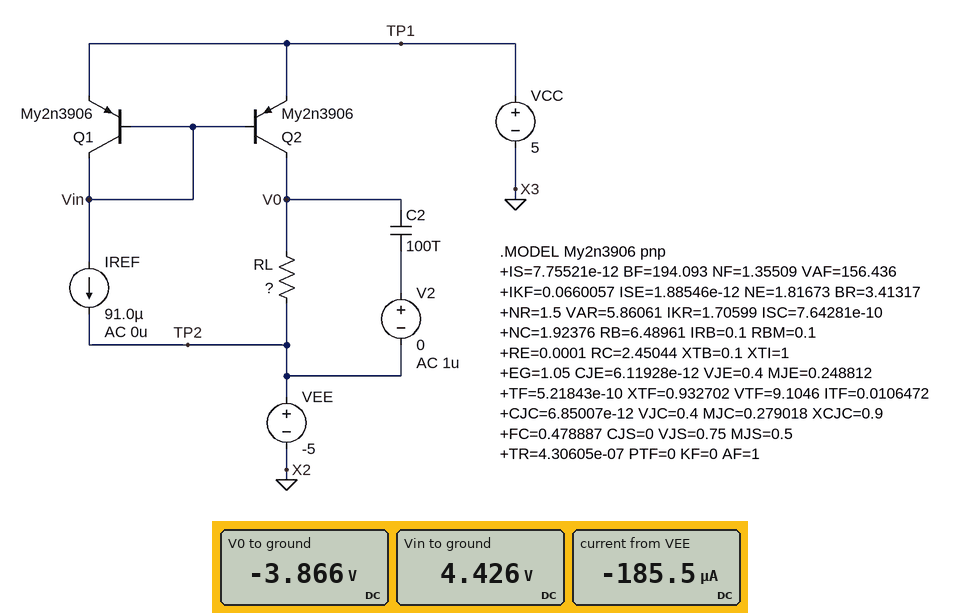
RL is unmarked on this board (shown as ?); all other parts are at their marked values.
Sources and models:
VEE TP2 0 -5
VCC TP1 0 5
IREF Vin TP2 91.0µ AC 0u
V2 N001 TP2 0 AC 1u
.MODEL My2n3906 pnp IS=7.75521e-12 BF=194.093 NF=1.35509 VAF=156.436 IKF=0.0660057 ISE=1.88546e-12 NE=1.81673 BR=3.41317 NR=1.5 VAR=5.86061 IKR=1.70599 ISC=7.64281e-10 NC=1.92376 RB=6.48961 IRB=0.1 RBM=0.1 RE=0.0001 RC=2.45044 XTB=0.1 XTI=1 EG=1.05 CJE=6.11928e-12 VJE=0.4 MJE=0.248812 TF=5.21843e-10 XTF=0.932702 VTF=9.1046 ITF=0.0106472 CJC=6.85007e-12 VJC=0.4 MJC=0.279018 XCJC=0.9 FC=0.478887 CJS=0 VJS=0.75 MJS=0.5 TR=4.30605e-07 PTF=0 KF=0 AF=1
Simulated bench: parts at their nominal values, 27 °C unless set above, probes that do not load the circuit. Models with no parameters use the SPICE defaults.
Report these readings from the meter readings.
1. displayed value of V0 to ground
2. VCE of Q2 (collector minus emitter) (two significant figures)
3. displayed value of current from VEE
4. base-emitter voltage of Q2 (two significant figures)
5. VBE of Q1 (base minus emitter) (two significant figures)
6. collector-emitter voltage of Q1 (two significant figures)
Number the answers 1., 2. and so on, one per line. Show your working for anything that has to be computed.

1. -3.866 V
2. -3.866 V - 5 V = -8.9 V
3. -185.5 µA
4. 4.426 V - 5 V = -570 mV
5. 4.426 V - 5 V = -570 mV
6. 4.426 V - 5 V = -570 mV
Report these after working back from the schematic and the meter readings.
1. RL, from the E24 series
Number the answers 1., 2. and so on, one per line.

1. 12 kΩ
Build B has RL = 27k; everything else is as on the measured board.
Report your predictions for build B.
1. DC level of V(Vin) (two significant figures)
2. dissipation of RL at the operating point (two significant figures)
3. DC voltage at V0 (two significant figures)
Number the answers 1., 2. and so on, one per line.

1. 4.4 V
2. 240 µW
3. -2.5 V
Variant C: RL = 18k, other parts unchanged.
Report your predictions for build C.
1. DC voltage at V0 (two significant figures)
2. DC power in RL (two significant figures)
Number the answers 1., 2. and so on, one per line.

1. -3.3 V
2. 160 µW
